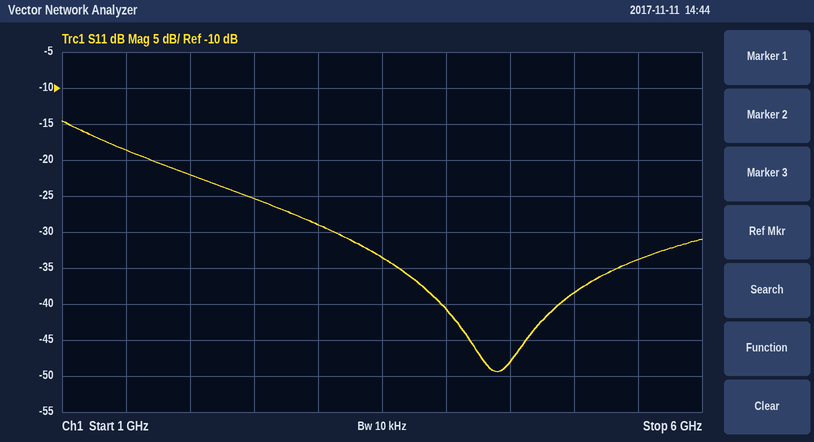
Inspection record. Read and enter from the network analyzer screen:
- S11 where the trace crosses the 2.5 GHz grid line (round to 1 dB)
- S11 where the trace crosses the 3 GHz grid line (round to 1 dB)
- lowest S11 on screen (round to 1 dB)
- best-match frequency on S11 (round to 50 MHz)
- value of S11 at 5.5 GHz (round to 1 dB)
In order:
-25 dB
-29 dB
-49 dB
4.40 GHz
-34 dB
